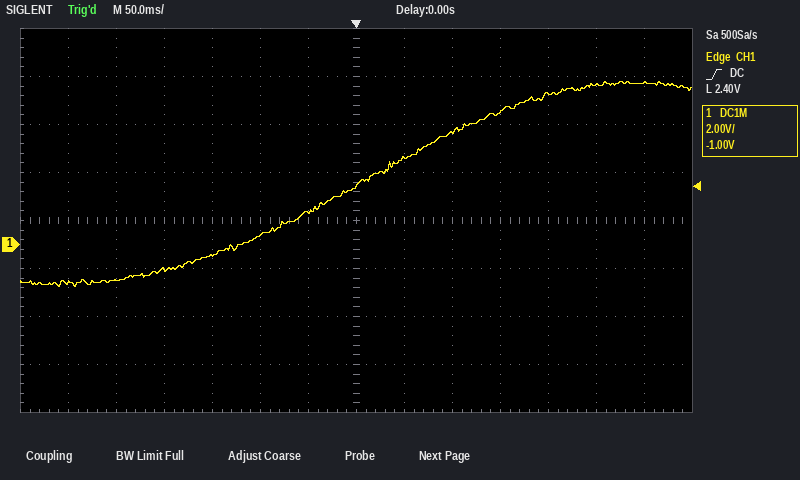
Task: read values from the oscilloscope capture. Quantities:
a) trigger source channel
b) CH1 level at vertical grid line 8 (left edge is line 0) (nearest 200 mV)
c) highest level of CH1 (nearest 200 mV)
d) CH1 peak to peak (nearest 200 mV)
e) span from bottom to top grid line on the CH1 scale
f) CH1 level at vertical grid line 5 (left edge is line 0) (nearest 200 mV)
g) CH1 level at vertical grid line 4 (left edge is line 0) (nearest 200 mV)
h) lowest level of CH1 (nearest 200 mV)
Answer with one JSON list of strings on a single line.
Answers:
["CH1", "3.6 V", "6.8 V", "8.6 V", "16 V", "400 mV", "-400 mV", "-1.8 V"]
